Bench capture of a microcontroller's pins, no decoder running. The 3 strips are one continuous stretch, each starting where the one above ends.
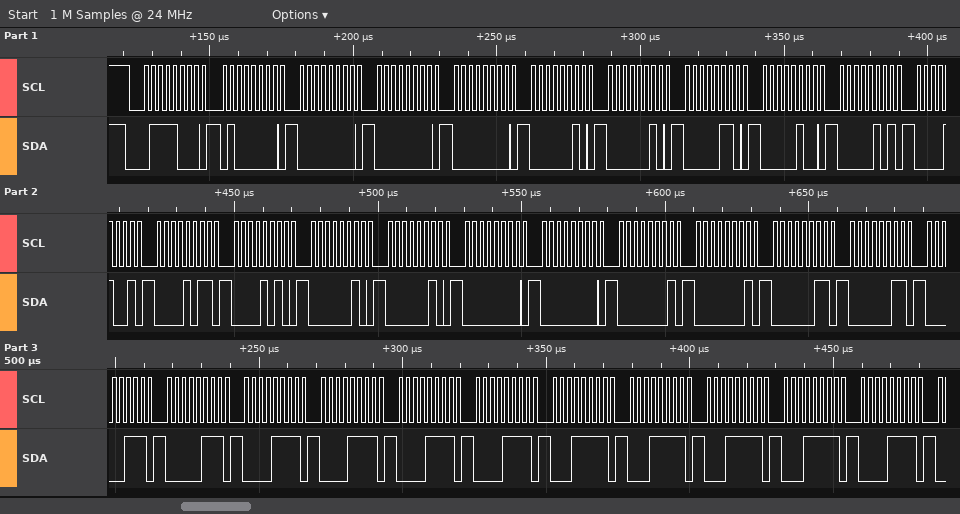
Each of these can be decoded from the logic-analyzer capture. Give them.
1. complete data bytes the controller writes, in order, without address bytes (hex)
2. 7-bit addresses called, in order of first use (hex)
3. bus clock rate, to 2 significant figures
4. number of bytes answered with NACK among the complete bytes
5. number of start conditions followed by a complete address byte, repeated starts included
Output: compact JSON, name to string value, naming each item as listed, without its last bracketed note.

{"complete data bytes the controller writes, in order, without address bytes": "40 00 00 00 02 02 06 04 05 09 0B 0A 02 02 00 00 01 01 03 03 07 07 0F 0F 0F 0F 1F 1F 1F 1F 0F", "7-bit addresses called, in order of first use": "0x3C", "bus clock rate, to 2 significant figures": "400 kHz", "number of bytes answered with NACK among the complete bytes": "0", "number of start conditions followed by a complete address byte, repeated starts included": "1"}
